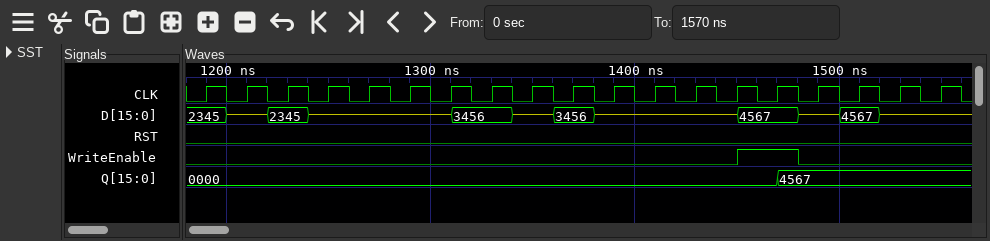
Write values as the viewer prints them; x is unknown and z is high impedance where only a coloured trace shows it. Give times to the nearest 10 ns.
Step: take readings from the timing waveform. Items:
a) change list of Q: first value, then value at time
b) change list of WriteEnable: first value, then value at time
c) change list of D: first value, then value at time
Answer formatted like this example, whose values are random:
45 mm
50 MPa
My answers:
0000, 4567 at 1470 ns
0, 1 at 1450 ns, 0 at 1480 ns
2345, z at 1200 ns, 2345 at 1220 ns, z at 1240 ns, 3456 at 1310 ns, z at 1340 ns, 3456 at 1360 ns, z at 1380 ns, 4567 at 1450 ns, z at 1480 ns, 4567 at 1500 ns, z at 1520 ns
